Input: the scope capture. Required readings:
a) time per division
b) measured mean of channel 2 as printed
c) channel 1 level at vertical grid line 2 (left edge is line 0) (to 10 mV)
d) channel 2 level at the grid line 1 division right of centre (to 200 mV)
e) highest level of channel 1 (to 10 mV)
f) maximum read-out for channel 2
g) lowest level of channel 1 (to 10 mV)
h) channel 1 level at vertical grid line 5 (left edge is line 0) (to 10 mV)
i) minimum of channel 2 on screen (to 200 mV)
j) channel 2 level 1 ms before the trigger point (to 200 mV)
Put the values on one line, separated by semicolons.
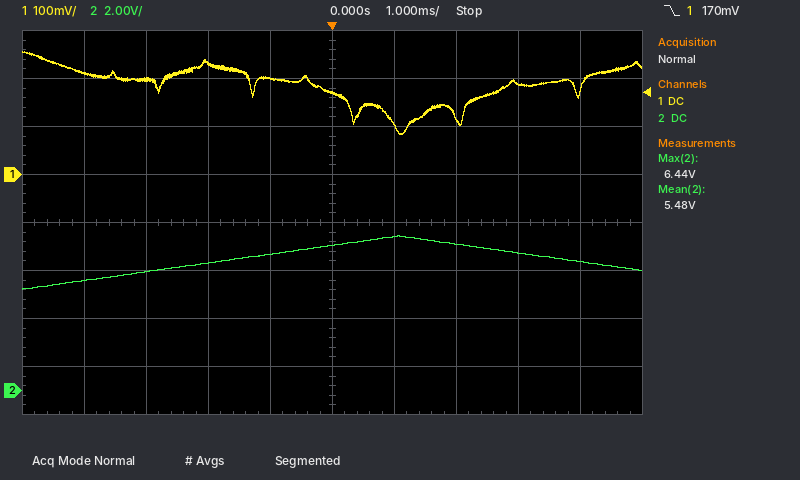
1 ms; 5.48 V; 200 mV; 6.4 V; 260 mV; 6.44 V; 80 mV; 170 mV; 4.2 V; 5.6 V
